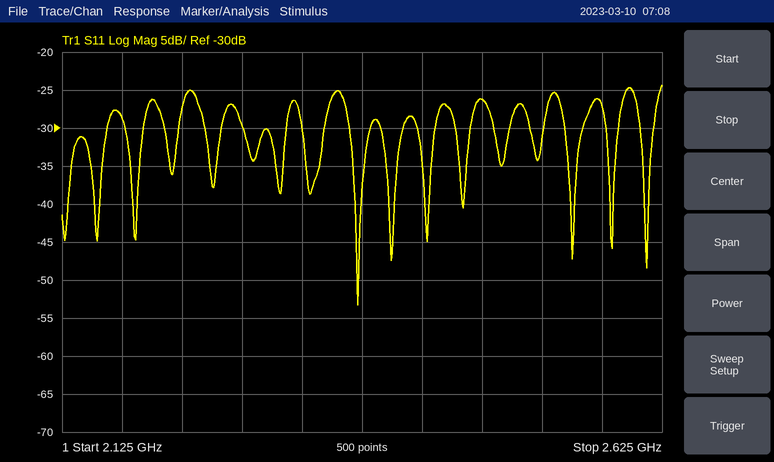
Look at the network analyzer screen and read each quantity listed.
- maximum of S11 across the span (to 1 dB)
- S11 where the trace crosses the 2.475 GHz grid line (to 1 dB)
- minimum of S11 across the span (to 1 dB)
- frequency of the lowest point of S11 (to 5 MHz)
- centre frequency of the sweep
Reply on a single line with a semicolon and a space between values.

-24 dB; -26 dB; -53 dB; 2.370 GHz; 2.375 GHz
